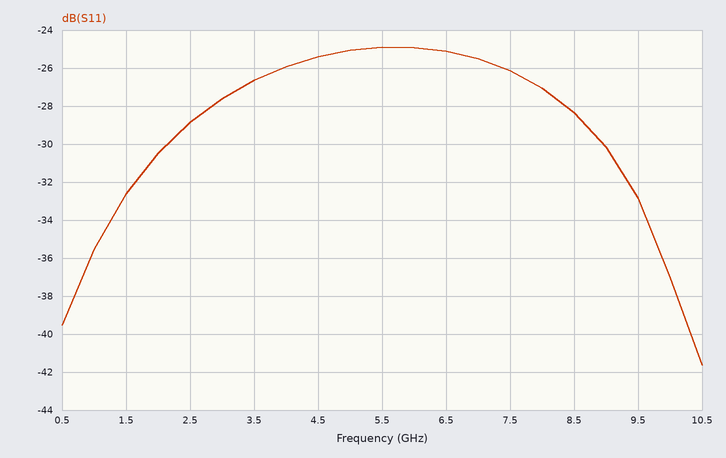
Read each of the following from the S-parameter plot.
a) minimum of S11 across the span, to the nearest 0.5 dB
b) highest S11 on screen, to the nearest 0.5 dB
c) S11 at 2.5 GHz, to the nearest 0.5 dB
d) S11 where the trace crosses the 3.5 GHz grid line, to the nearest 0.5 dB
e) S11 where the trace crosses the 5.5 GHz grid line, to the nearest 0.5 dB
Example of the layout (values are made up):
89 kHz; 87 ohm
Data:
-41.5 dB; -25.0 dB; -29.0 dB; -26.5 dB; -25.0 dB
